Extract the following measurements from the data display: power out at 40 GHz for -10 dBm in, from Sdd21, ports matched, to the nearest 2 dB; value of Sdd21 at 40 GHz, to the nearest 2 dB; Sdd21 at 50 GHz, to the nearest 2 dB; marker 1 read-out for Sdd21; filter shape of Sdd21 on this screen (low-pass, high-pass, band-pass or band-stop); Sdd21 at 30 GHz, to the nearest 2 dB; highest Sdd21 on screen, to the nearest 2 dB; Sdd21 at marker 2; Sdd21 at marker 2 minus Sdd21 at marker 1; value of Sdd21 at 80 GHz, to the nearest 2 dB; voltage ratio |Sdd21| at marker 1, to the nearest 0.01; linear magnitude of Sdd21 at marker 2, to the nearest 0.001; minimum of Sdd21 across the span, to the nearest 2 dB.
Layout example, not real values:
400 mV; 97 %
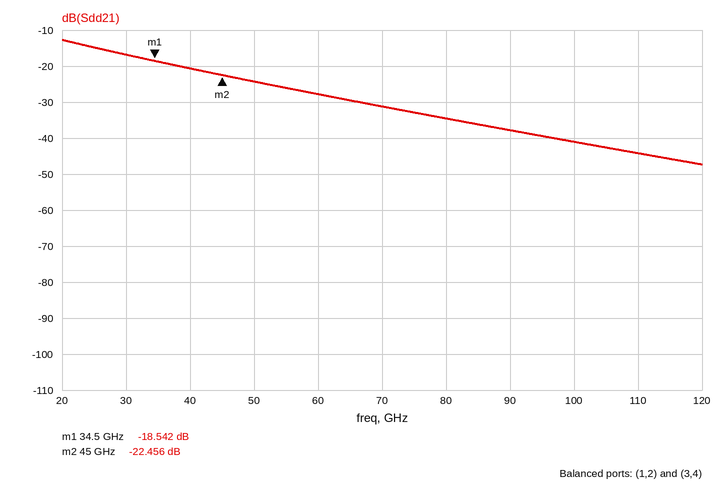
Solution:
-30 dBm; -20 dB; -24 dB; -18.542 dB; low-pass; -16 dB; -12 dB; -22.456 dB; -3.914 dB; -34 dB; 0.12; 0.075; -48 dB
